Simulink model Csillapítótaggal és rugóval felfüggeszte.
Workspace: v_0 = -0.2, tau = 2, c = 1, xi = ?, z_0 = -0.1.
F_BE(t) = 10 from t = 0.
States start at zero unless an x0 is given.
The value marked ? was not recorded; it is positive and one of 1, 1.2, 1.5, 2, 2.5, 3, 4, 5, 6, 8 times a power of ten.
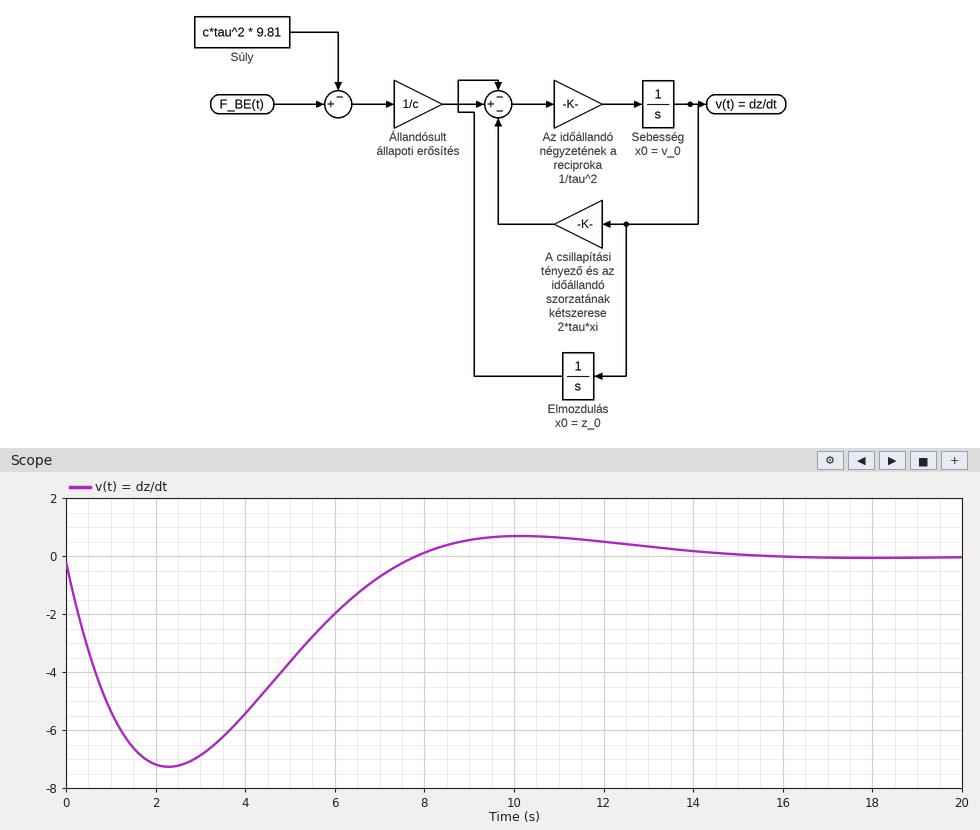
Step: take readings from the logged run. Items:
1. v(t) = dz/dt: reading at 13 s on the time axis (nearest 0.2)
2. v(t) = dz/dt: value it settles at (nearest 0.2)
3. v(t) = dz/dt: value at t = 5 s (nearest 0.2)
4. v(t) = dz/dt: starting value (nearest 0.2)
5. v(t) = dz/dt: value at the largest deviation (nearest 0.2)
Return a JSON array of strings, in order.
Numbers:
["0.4", "0.0", "-3.6", "-0.2", "-7.2"]
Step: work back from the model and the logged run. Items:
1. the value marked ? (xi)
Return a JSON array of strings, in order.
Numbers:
["0.6"]
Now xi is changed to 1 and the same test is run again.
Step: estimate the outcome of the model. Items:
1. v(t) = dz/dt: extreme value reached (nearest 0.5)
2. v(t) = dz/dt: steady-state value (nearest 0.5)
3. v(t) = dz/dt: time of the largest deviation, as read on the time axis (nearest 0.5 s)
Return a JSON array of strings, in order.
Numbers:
["-5.5", "0.0", "2.0 s"]
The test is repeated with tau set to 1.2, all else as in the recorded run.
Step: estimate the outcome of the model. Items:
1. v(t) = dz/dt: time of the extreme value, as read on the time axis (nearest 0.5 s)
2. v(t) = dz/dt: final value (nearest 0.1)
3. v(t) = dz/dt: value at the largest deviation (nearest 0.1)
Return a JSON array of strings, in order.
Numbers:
["1.5 s", "0.0", "-1.7"]
